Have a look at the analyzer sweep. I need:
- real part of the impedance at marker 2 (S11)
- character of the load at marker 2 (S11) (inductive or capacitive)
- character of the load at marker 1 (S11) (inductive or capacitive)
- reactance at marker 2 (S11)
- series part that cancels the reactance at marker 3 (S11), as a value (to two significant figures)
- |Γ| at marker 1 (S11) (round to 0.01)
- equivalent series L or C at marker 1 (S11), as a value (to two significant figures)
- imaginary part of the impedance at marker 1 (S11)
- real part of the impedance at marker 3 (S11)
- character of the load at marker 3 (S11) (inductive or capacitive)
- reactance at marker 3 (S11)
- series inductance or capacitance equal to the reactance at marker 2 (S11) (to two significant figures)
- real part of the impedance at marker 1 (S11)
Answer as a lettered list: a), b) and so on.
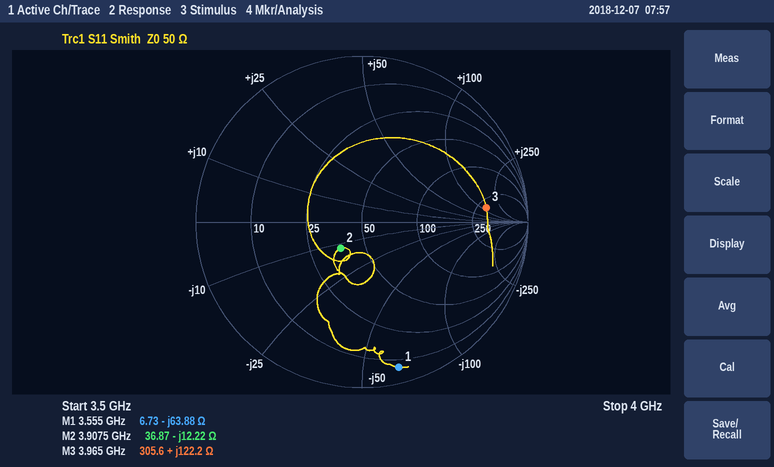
a) 36.87 Ω
b) capacitive
c) capacitive
d) -12.22 Ω
e) 330 fF
f) 0.90
g) 700 fF
h) -63.88 Ω
i) 305.6 Ω
j) inductive
k) +122.2 Ω
l) 3.3 pF
m) 6.73 Ω
